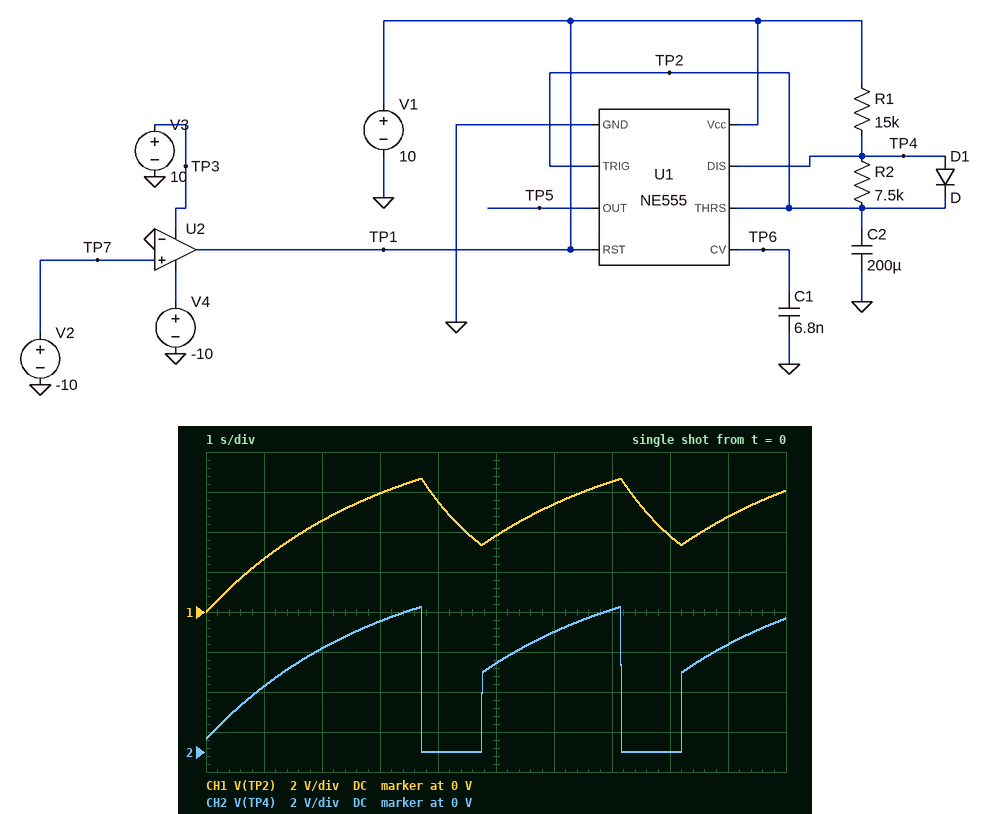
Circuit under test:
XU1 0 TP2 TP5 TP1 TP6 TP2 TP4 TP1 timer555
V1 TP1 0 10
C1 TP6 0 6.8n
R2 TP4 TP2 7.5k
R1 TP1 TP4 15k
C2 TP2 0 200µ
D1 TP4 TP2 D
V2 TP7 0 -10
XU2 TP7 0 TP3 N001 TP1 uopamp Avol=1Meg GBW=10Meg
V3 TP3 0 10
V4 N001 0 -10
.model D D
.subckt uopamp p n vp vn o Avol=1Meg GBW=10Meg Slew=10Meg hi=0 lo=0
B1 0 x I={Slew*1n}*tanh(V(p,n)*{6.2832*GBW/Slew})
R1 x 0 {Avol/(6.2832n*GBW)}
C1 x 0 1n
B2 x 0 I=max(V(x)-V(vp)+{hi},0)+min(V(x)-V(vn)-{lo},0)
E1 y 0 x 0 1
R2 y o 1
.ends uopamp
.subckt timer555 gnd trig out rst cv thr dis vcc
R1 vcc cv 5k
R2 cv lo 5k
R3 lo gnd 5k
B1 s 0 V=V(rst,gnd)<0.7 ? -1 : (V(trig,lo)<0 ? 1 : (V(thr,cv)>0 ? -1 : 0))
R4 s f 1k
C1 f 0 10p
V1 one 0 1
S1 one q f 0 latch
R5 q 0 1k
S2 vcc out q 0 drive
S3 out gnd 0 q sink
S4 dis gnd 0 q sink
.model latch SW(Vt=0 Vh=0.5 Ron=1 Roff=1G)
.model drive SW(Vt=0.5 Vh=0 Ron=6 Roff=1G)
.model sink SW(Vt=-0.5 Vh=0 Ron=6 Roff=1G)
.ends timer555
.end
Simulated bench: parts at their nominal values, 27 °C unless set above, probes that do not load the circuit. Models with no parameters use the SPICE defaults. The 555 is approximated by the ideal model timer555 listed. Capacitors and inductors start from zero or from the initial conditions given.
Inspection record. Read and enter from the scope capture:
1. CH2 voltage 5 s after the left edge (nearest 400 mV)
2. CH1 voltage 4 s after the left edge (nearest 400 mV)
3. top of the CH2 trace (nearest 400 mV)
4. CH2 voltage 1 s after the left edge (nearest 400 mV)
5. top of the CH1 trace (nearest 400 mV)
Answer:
4.4 V
5.6 V
7.2 V
3.2 V
6.8 V
